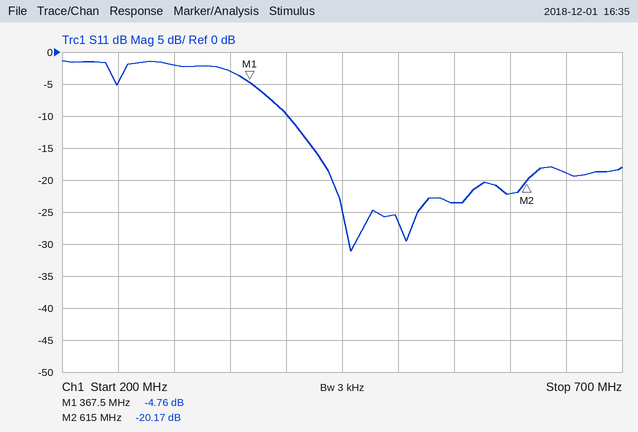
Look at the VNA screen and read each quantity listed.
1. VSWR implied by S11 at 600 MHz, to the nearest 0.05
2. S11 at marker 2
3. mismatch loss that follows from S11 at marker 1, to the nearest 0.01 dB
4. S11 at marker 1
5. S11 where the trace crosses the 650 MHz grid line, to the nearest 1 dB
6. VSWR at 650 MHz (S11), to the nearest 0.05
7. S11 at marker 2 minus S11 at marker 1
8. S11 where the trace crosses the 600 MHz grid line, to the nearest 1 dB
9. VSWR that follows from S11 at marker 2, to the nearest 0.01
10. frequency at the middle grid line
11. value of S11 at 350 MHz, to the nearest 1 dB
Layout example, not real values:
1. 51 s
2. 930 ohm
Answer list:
1. 1.15
2. -20.17 dB
3. 1.77 dB
4. -4.76 dB
5. -19 dB
6. 1.25
7. -15.41 dB
8. -22 dB
9. 1.22
10. 450 MHz
11. -3 dB
